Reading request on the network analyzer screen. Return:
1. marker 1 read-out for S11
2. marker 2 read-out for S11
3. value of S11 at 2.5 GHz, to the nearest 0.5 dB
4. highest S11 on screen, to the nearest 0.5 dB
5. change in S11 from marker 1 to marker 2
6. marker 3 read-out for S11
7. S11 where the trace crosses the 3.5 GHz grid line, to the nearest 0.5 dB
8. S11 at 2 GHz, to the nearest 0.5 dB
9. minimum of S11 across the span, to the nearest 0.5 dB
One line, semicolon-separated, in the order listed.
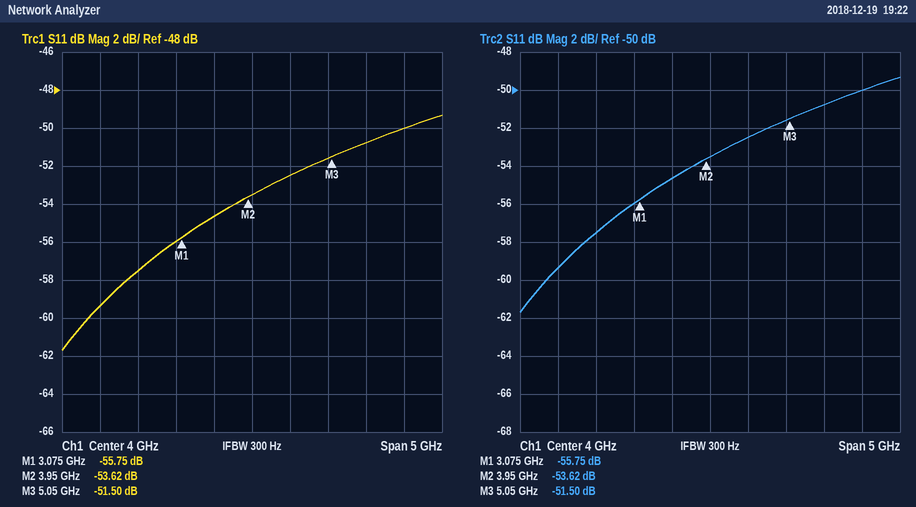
-55.75 dB; -53.62 dB; -57.5 dB; -49.5 dB; 2.13 dB; -51.50 dB; -54.5 dB; -59.5 dB; -61.5 dB
